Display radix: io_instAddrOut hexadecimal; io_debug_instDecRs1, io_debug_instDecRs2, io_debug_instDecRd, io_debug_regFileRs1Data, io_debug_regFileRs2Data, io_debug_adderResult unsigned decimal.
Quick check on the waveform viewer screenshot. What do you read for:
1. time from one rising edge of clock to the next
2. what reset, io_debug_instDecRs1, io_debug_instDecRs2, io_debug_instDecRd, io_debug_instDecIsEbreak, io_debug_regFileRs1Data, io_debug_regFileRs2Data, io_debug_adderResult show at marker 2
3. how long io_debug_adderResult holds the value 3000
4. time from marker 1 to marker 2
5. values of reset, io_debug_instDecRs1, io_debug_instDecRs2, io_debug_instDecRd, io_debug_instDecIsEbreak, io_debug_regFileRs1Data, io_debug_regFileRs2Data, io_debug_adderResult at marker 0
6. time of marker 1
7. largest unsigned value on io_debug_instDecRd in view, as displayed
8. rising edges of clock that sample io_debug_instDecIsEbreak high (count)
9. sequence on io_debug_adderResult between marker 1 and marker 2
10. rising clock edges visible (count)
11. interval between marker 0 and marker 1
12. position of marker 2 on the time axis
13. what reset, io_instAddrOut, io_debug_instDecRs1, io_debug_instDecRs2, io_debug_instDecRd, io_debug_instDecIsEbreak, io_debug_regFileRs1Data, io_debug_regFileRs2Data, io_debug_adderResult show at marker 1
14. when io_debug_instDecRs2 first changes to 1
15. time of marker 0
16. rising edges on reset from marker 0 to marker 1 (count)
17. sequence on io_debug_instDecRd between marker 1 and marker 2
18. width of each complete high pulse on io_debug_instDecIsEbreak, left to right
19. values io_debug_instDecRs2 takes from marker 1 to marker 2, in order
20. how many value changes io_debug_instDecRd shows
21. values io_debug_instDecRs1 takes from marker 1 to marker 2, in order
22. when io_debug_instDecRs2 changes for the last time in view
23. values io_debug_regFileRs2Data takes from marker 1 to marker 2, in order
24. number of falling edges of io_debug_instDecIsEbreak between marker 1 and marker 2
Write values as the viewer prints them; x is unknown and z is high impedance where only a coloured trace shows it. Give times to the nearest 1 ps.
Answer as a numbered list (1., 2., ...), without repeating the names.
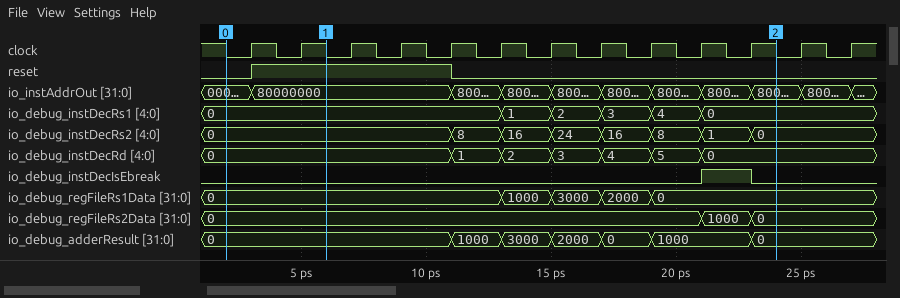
1. 2 ps
2. reset=0, io_debug_instDecRs1=0, io_debug_instDecRs2=0, io_debug_instDecRd=0, io_debug_instDecIsEbreak=0, io_debug_regFileRs1Data=0, io_debug_regFileRs2Data=0, io_debug_adderResult=0
3. 2 ps
4. 18 ps
5. reset=0, io_debug_instDecRs1=0, io_debug_instDecRs2=0, io_debug_instDecRd=0, io_debug_instDecIsEbreak=0, io_debug_regFileRs1Data=0, io_debug_regFileRs2Data=0, io_debug_adderResult=0
6. 6 ps
7. 5
8. 1
9. 0, 1000, 3000, 2000, 0, 1000, 0
10. 13
11. 4 ps
12. 24 ps
13. reset=1, io_instAddrOut=80000000, io_debug_instDecRs1=0, io_debug_instDecRs2=0, io_debug_instDecRd=0, io_debug_instDecIsEbreak=0, io_debug_regFileRs1Data=0, io_debug_regFileRs2Data=0, io_debug_adderResult=0
14. 21 ps
15. 2 ps
16. 1
17. 0, 1, 2, 3, 4, 5, 0
18. 2 ps
19. 0, 8, 16, 24, 16, 8, 1, 0
20. 6
21. 0, 1, 2, 3, 4, 0
22. 23 ps
23. 0, 1000, 0
24. 1
